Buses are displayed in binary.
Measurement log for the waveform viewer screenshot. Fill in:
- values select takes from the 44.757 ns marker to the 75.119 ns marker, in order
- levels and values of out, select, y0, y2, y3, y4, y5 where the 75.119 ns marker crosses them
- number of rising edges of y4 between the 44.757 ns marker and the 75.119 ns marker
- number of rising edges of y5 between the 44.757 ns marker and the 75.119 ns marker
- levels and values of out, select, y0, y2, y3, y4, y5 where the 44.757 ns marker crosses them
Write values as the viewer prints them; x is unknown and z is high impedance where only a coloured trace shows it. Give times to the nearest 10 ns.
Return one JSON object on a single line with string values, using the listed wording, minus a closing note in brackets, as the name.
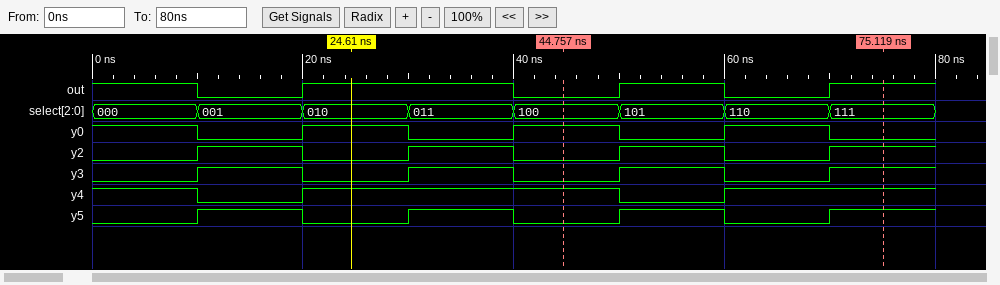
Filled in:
{"values select takes from the 44.757 ns marker to the 75.119 ns marker, in order": "100, 101, 110, 111", "levels and values of out, select, y0, y2, y3, y4, y5 where the 75.119 ns marker crosses them": "out=1, select=111, y0=0, y2=1, y3=1, y4=1, y5=1", "number of rising edges of y4 between the 44.757 ns marker and the 75.119 ns marker": "1", "number of rising edges of y5 between the 44.757 ns marker and the 75.119 ns marker": "2", "levels and values of out, select, y0, y2, y3, y4, y5 where the 44.757 ns marker crosses them": "out=0, select=100, y0=1, y2=0, y3=0, y4=1, y5=0"}
